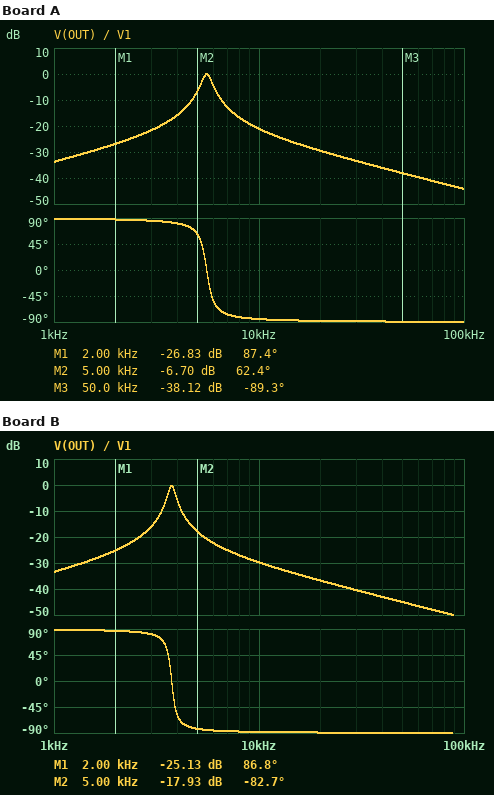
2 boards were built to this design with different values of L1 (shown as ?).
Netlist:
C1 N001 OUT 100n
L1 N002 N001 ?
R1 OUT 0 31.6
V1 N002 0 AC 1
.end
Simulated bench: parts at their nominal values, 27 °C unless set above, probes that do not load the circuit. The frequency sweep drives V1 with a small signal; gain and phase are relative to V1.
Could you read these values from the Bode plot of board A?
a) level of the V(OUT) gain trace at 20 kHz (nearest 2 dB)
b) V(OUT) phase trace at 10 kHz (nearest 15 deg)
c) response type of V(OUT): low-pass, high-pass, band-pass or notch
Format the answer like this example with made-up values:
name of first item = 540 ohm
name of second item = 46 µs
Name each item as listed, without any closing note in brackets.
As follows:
level of the V(OUT) gain trace at 20 kHz = -30 dB
V(OUT) phase trace at 10 kHz = -90 deg
response type of V(OUT): low-pass, high-pass, band-pass or notch = band-pass
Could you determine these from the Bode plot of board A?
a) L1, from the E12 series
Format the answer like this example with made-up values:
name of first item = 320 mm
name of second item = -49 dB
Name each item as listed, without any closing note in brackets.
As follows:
L1, from the E12 series = 8.2 mH
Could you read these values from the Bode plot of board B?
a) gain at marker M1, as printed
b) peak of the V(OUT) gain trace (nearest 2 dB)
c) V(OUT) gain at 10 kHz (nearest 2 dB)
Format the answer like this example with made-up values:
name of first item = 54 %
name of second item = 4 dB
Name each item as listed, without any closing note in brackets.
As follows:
gain at marker M1, as printed = -25.13 dB
peak of the V(OUT) gain trace = 0 dB
V(OUT) gain at 10 kHz = -30 dB
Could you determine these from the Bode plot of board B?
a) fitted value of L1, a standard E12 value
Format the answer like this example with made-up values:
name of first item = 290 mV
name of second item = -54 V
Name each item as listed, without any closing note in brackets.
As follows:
fitted value of L1, a standard E12 value = 18 mH
